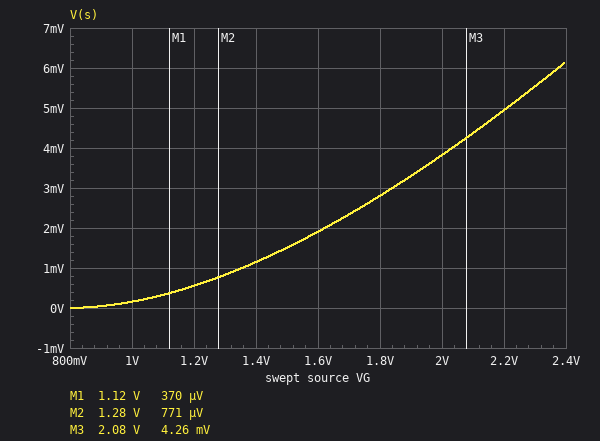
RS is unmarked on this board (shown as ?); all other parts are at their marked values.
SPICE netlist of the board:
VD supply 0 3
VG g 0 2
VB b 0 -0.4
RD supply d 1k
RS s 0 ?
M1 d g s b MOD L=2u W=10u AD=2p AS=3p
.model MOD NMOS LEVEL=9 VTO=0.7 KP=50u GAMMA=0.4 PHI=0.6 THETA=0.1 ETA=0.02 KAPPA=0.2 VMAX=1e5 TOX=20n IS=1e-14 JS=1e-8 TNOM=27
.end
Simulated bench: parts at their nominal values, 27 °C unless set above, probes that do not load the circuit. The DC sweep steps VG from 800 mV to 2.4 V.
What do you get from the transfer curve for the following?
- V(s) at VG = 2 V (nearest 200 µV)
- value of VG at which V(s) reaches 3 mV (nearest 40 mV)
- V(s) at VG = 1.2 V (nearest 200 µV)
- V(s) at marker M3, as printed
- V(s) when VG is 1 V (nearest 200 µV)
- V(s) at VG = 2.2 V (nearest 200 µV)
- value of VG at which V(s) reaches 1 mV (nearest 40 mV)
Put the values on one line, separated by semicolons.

3.8 mV; 1.84 V; 600 µV; 4.26 mV; 200 µV; 5.0 mV; 1.36 V
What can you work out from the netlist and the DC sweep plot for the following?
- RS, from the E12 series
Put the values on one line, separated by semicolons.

33 Ω
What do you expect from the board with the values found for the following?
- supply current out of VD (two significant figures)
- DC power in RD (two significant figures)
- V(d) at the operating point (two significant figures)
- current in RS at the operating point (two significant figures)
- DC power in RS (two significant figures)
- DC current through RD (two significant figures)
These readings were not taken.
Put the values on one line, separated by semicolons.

120 µA; 13 µW; 2.9 V; 120 µA; 440 nW; 120 µA
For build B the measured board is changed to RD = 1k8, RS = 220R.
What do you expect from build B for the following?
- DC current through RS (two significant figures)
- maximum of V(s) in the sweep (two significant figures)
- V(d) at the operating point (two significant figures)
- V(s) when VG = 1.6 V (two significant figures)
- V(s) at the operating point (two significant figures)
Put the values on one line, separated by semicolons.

110 µA; 39 mV; 2.8 V; 12 mV; 25 mV
